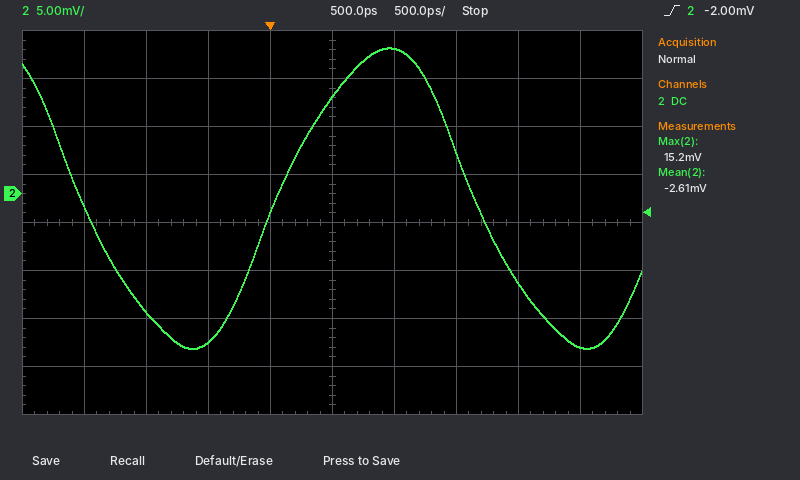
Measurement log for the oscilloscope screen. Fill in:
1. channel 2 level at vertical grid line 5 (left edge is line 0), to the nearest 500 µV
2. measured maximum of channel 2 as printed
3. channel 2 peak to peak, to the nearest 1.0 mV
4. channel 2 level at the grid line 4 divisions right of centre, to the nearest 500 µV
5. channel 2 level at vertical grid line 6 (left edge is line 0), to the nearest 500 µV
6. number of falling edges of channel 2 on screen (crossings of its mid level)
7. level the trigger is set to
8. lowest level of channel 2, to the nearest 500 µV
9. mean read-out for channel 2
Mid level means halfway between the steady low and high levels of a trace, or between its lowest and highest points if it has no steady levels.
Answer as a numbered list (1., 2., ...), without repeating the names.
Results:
1. 10.0 mV
2. 15.2 mV
3. 31.0 mV
4. -16.0 mV
5. 15.0 mV
6. 2
7. -2.00 mV
8. -16.0 mV
9. -2.61 mV
